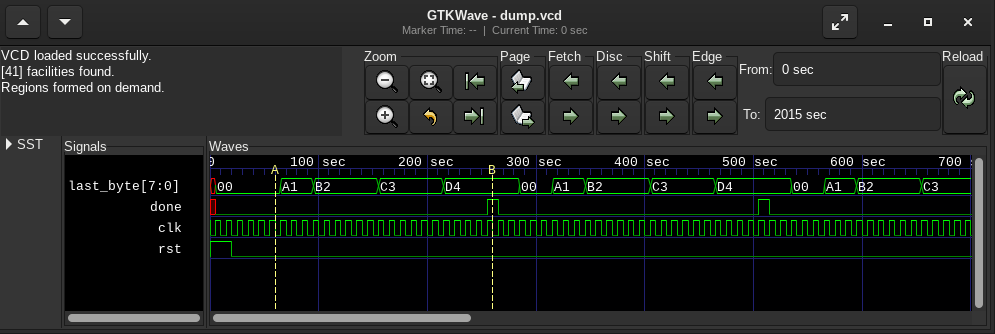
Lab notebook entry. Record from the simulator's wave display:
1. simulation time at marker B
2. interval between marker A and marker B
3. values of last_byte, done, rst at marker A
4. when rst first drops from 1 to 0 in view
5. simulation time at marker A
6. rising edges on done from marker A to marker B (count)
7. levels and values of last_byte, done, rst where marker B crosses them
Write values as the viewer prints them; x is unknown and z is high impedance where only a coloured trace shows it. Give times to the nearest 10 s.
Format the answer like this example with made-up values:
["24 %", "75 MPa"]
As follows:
["260 s", "200 s", "last_byte=00, done=0, rst=0", "20 s", "60 s", "1", "last_byte=D4, done=1, rst=0"]
